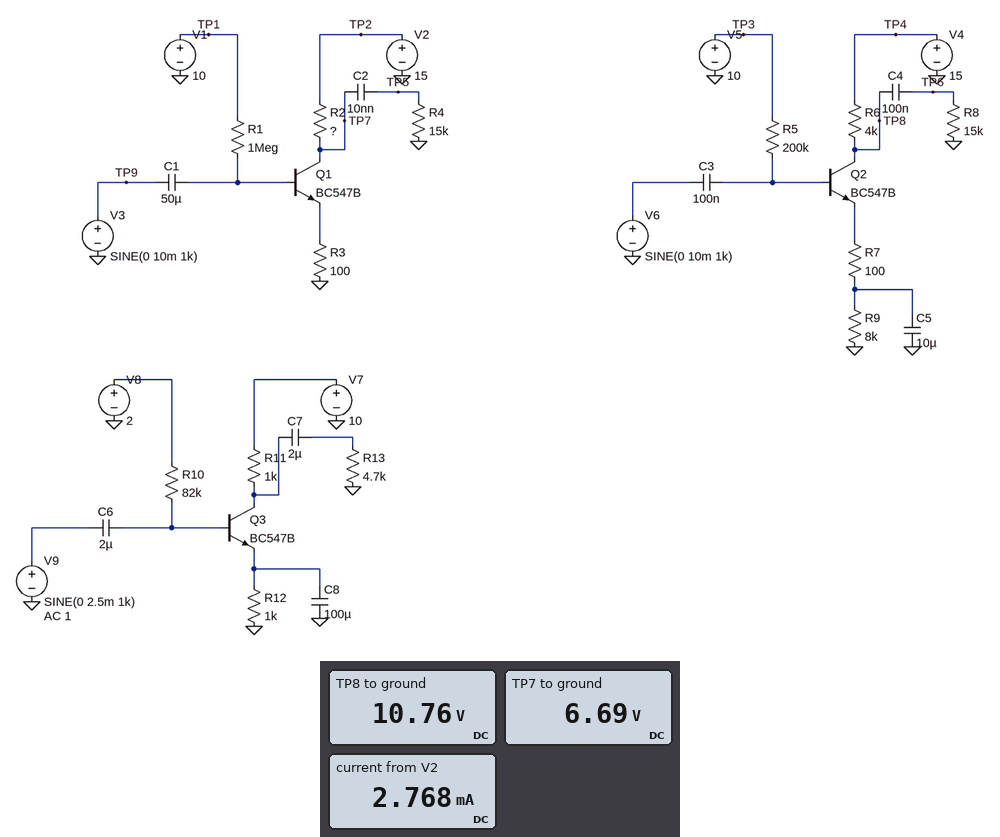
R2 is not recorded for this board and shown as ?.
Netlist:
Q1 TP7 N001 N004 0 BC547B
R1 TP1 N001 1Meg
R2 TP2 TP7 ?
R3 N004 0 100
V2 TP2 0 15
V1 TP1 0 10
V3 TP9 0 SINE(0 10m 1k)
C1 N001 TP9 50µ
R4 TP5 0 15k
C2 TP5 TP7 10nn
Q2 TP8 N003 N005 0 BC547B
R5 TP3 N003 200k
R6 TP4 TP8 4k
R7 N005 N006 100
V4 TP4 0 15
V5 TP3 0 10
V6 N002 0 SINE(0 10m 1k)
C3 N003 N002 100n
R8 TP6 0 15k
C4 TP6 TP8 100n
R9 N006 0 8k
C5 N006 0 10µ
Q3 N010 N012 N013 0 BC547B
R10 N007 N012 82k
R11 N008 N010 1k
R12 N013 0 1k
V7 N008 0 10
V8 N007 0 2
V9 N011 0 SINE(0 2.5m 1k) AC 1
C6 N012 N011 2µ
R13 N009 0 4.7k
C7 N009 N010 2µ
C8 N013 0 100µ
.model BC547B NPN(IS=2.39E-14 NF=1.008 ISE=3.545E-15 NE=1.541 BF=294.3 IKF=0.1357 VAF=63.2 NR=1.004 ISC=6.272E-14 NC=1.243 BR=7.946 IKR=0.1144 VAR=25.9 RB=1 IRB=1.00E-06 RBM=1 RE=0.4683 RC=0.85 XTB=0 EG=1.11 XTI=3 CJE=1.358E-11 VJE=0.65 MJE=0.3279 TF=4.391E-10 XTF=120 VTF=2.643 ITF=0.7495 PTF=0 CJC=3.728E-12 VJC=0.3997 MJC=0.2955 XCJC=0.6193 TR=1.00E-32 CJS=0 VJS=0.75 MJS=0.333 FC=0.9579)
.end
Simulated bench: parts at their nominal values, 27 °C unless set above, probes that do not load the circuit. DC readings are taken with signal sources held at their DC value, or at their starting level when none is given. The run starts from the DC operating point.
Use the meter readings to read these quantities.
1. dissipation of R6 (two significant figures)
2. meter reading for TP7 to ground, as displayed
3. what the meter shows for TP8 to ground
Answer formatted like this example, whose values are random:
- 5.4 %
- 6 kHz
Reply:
- 4.5 mW
- 6.69 V
- 10.76 V
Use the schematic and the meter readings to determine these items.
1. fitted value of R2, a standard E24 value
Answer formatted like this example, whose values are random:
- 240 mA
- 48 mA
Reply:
- 3 kΩ
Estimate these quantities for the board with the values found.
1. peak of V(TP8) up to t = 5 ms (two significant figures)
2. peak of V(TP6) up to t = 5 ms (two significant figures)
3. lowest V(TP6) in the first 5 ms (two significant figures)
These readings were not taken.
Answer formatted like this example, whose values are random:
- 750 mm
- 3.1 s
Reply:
- 11 V
- 270 mV
- -250 mV
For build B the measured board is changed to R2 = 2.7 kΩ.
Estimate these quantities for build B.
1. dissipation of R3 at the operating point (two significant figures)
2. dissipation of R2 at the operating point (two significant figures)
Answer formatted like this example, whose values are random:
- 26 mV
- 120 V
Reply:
- 790 µW
- 21 mW
